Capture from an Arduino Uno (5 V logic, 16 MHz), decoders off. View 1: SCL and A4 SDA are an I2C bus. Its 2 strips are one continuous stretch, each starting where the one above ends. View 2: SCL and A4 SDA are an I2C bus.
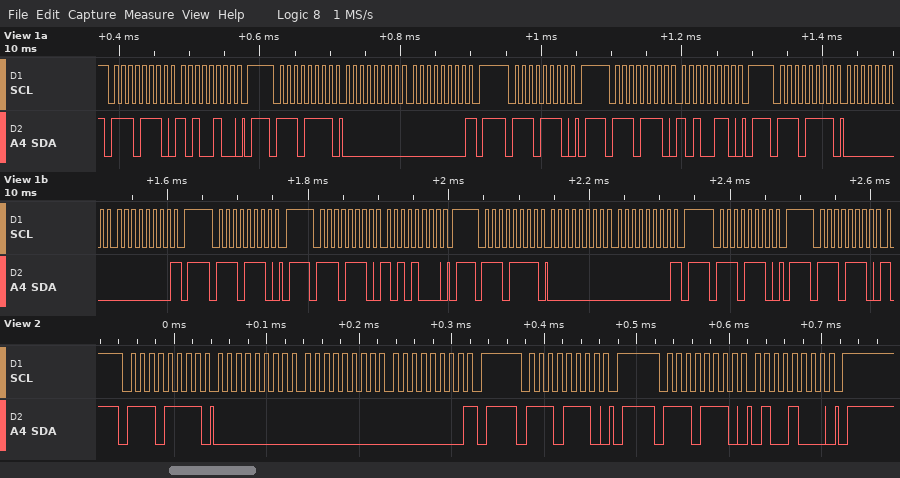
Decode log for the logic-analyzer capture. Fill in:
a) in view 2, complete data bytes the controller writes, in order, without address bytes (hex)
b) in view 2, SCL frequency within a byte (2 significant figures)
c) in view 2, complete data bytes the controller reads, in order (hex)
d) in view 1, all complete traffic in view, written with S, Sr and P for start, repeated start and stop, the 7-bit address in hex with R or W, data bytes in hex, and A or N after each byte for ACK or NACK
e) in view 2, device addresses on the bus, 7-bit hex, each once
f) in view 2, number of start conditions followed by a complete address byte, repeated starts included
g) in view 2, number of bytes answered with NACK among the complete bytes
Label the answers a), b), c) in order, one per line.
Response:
a) 48
b) 100 kHz
c) 00 00 00
d) S 77W A A4 A P S 77R A 00 A 00 N P S 77W A P S 77W A A6 A P S 77R A 00 A 00 N P S 77W A P S 77W A A8 A P S 77R A 00 A 00 N P S 77W A P S 77W A
e) 0x77
f) 3
g) 1
